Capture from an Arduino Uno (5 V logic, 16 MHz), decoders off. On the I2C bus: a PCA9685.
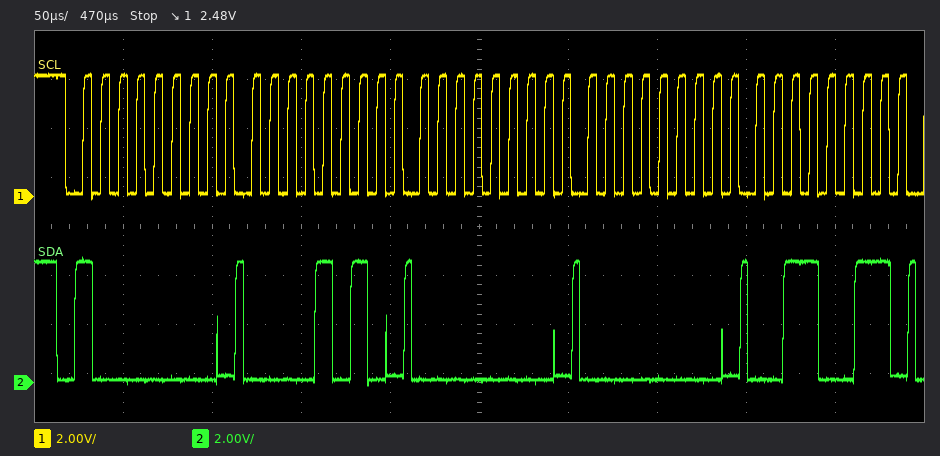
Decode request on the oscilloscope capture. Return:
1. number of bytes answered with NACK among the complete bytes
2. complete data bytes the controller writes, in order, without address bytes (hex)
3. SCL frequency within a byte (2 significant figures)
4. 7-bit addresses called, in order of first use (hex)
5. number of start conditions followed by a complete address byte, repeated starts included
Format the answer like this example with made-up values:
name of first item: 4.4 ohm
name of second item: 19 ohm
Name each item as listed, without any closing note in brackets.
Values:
number of bytes answered with NACK among the complete bytes: 0
complete data bytes the controller writes, in order, without address bytes: 0A 00 00 33
SCL frequency within a byte: 100 kHz
7-bit addresses called, in order of first use: 0x40
number of start conditions followed by a complete address byte, repeated starts included: 1
